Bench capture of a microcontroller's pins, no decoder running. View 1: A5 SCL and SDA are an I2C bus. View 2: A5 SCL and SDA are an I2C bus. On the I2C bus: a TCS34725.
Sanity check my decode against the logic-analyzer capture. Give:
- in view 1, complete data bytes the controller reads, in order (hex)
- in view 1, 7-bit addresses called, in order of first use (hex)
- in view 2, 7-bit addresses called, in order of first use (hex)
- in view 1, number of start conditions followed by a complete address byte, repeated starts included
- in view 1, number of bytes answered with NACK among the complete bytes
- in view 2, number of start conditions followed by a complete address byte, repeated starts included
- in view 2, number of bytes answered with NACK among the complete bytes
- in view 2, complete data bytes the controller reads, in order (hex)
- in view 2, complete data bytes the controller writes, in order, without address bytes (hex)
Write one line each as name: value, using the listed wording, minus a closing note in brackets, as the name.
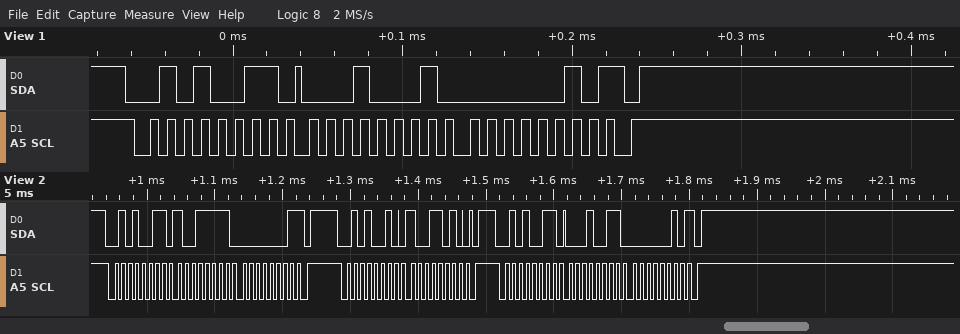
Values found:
in view 1, complete data bytes the controller reads, in order: 11 02
in view 1, 7-bit addresses called, in order of first use: 0x29
in view 2, 7-bit addresses called, in order of first use: 0x29
in view 1, number of start conditions followed by a complete address byte, repeated starts included: 1
in view 1, number of bytes answered with NACK among the complete bytes: 1
in view 2, number of start conditions followed by a complete address byte, repeated starts included: 3
in view 2, number of bytes answered with NACK among the complete bytes: 2
in view 2, complete data bytes the controller reads, in order: 9F 01 13 02
in view 2, complete data bytes the controller writes, in order, without address bytes: 9A
